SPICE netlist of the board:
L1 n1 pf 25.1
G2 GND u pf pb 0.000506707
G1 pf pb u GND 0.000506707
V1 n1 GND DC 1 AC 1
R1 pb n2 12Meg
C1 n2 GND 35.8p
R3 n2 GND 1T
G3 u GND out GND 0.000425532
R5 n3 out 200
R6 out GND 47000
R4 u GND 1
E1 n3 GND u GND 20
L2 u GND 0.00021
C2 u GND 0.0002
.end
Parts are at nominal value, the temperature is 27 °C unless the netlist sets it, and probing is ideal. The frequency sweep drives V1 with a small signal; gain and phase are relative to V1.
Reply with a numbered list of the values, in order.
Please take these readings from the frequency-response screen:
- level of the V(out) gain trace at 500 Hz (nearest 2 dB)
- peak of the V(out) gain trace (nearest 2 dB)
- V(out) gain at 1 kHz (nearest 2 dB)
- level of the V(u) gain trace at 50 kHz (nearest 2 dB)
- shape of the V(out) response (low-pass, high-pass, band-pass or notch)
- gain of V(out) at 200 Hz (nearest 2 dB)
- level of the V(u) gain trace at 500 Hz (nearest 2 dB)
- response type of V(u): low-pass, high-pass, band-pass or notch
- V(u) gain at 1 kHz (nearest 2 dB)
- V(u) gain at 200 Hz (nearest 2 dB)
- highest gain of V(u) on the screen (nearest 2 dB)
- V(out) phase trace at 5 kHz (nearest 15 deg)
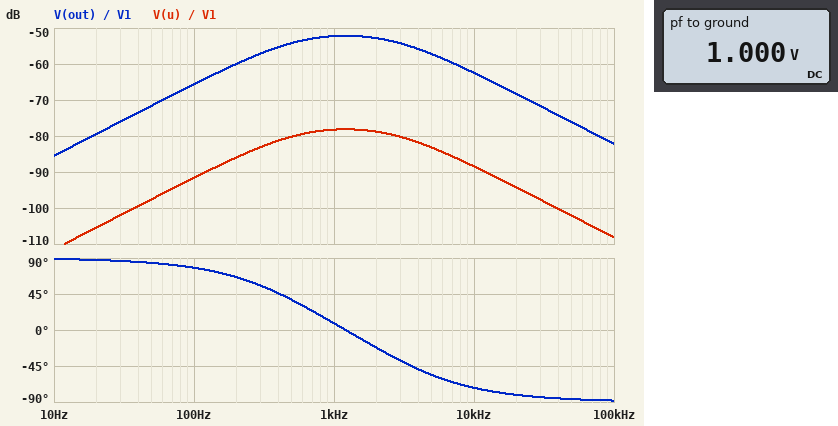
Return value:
1. -54 dB
2. -52 dB
3. -52 dB
4. -102 dB
5. band-pass
6. -60 dB
7. -80 dB
8. band-pass
9. -78 dB
10. -86 dB
11. -78 dB
12. -60 deg
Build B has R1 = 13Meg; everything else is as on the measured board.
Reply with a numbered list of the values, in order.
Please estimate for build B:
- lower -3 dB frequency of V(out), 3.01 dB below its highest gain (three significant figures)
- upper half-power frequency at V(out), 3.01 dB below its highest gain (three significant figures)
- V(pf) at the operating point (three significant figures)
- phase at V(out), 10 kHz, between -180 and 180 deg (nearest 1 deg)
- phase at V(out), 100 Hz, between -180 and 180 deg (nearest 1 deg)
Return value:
1. 391 Hz
2. 3.74 kHz
3. 1.00 V
4. -71 deg
5. 77 deg
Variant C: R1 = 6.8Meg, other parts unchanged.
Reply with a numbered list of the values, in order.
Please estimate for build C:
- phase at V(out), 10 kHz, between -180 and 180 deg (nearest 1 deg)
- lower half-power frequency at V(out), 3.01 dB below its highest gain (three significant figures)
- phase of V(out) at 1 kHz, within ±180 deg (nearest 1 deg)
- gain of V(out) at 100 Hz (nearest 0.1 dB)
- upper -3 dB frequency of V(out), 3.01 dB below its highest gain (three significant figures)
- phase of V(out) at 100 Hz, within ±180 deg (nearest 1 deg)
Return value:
1. -78 deg
2. 548 Hz
3. 12 deg
4. -65.5 dB
5. 2.67 kHz
6. 82 deg
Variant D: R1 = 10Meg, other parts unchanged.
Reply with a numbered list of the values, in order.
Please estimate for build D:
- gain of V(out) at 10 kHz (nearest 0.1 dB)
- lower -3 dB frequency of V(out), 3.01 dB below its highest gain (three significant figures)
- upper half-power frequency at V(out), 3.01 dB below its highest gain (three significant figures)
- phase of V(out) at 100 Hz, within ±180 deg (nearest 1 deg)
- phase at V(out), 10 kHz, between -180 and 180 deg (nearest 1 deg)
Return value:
1. -62.4 dB
2. 456 Hz
3. 3.21 kHz
4. 79 deg
5. -74 deg
